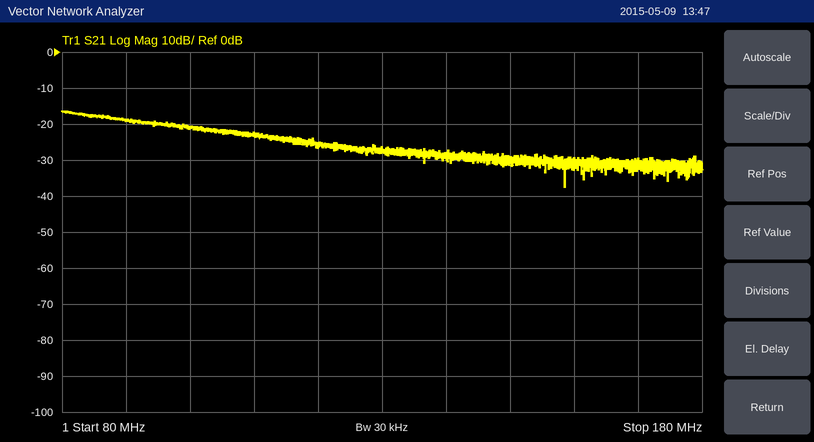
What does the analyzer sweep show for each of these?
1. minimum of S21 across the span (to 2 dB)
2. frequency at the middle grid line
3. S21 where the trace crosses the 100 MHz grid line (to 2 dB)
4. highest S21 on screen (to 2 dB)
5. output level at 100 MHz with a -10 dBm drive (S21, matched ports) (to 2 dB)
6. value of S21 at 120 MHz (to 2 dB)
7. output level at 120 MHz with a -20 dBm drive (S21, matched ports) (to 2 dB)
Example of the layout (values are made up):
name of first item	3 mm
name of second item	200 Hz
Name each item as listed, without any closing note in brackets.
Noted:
minimum of S21 across the span	-38 dB
frequency at the middle grid line	130 MHz
S21 where the trace crosses the 100 MHz grid line	-20 dB
highest S21 on screen	-16 dB
output level at 100 MHz with a -10 dBm drive (S21, matched ports)	-30 dBm
value of S21 at 120 MHz	-26 dB
output level at 120 MHz with a -20 dBm drive (S21, matched ports)	-46 dBm
